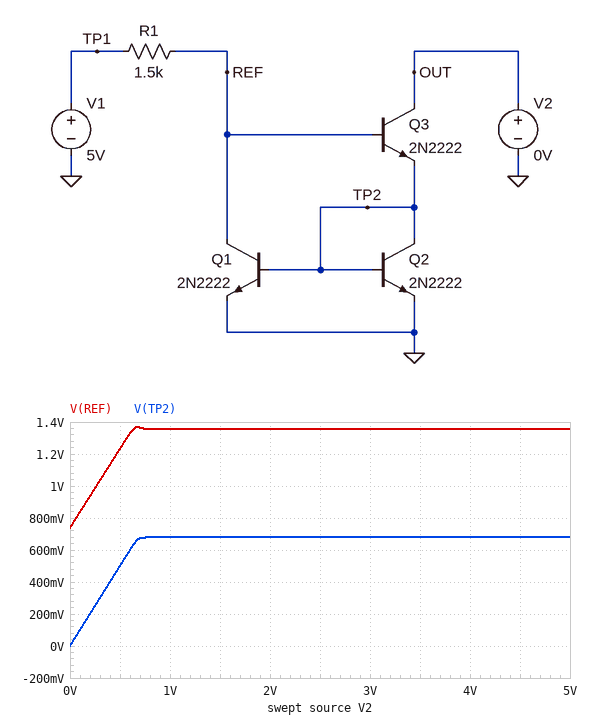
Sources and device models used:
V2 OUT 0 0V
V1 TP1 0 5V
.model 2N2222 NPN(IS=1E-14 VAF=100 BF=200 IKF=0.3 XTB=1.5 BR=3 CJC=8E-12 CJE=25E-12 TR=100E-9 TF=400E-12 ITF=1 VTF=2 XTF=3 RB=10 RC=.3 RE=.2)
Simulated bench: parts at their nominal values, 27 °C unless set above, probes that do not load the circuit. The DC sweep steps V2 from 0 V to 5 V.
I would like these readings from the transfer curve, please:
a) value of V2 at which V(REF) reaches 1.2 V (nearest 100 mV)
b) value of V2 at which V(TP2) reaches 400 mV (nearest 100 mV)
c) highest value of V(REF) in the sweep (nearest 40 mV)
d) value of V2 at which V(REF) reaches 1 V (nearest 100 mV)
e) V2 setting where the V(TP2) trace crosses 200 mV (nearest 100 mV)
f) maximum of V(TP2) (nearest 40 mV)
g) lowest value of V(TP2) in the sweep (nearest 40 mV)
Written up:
500 mV
400 mV
1.36 V
300 mV
200 mV
680 mV
0 V
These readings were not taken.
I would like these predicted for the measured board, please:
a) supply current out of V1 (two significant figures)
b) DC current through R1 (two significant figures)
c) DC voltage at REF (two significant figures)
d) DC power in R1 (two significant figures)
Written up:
2.8 mA
2.8 mA
740 mV
12 mW
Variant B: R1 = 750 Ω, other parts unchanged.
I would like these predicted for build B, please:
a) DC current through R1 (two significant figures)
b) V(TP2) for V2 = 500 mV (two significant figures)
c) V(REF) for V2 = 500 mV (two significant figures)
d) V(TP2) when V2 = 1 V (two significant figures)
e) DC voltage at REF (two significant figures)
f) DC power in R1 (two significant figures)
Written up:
5.6 mA
500 mV
1.3 V
700 mV
790 mV
24 mW
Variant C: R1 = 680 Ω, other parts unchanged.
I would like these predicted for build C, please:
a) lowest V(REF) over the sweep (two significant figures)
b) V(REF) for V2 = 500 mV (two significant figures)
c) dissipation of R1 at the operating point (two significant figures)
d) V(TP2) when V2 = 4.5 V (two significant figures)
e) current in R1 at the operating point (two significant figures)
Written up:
790 mV
1.3 V
26 mW
700 mV
6.2 mA
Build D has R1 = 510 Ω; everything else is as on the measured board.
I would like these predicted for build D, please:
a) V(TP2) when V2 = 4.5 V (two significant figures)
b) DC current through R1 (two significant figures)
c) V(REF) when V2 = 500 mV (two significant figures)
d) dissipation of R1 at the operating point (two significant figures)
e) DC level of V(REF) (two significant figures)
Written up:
710 mV
8.2 mA
1.3 V
34 mW
820 mV
